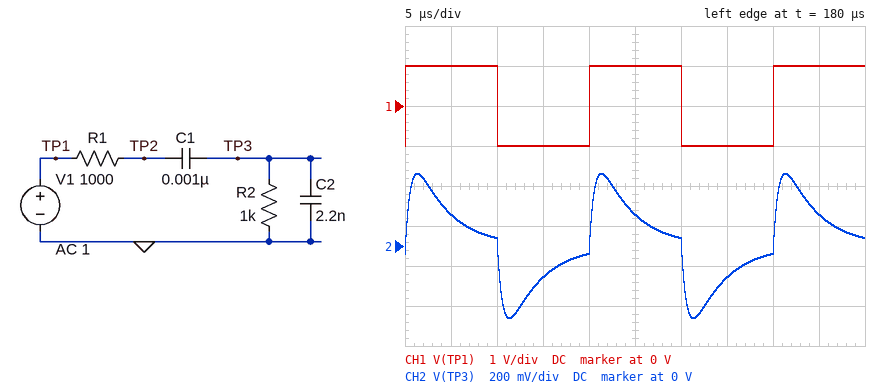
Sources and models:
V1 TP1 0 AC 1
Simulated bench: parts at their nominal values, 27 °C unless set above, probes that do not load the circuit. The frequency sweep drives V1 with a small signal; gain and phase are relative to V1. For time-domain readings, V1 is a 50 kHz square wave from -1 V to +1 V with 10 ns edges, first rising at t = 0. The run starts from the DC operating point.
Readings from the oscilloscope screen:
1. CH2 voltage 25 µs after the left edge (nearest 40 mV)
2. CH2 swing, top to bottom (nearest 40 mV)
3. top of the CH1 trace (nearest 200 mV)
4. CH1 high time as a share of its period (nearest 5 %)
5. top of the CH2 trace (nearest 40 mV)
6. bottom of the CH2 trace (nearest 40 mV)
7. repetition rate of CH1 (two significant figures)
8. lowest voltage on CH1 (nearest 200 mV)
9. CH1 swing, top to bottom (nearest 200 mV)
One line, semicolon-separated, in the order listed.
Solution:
160 mV; 720 mV; 1.0 V; 50 %; 360 mV; -360 mV; 50 kHz; -1.0 V; 2.0 V
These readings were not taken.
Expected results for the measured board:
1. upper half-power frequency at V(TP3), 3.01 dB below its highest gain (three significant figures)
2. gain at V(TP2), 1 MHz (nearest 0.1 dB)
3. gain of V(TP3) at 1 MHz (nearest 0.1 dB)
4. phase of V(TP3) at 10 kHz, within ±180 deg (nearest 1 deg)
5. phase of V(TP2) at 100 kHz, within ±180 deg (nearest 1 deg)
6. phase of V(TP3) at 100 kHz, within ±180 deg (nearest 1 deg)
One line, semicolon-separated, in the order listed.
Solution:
338 kHz; -13.0 dB; -23.1 dB; 75 deg; -24 deg; 3 deg
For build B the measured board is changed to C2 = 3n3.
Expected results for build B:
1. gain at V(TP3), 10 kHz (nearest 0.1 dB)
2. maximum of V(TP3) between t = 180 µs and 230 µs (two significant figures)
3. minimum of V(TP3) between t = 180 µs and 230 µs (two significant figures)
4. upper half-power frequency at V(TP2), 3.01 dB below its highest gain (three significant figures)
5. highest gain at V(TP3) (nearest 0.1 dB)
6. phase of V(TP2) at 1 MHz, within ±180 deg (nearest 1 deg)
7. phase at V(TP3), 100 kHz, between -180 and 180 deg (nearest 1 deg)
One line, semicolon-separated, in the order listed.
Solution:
-24.4 dB; 270 mV; -270 mV; 194 kHz; -14.5 dB; -78 deg; -5 deg
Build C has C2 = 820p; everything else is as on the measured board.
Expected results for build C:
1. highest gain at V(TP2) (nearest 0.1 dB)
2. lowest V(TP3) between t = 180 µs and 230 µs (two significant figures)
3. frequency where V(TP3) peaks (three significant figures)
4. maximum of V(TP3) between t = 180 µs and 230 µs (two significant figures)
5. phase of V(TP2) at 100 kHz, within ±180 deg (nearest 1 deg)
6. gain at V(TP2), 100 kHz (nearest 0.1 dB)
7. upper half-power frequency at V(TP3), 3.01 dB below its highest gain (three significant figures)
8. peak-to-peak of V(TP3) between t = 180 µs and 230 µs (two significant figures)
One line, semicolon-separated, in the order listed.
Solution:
0 dB; -580 mV; 176 kHz; 580 mV; -20 deg; -1.9 dB; 599 kHz; 1.2 V
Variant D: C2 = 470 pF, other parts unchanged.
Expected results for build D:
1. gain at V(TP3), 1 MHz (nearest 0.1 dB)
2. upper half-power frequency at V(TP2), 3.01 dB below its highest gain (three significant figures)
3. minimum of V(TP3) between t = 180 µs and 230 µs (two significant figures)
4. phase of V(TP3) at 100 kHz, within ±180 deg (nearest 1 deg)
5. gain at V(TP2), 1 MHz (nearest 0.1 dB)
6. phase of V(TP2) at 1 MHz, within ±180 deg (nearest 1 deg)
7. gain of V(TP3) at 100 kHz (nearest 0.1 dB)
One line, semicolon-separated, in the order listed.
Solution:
-11.4 dB; 155 kHz; -690 mV; 28 deg; -8.0 dB; -55 deg; -8.9 dB
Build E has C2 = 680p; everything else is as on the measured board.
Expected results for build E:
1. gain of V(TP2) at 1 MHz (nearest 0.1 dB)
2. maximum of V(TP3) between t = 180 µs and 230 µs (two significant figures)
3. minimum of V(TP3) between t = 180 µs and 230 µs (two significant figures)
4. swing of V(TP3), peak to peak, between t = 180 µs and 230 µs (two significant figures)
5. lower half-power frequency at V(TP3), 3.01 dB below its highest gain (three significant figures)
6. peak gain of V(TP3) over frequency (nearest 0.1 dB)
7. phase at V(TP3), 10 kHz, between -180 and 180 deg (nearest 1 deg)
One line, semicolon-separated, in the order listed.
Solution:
-9.3 dB; 620 mV; -620 mV; 1.2 V; 54.6 kHz; -8.6 dB; 80 deg
